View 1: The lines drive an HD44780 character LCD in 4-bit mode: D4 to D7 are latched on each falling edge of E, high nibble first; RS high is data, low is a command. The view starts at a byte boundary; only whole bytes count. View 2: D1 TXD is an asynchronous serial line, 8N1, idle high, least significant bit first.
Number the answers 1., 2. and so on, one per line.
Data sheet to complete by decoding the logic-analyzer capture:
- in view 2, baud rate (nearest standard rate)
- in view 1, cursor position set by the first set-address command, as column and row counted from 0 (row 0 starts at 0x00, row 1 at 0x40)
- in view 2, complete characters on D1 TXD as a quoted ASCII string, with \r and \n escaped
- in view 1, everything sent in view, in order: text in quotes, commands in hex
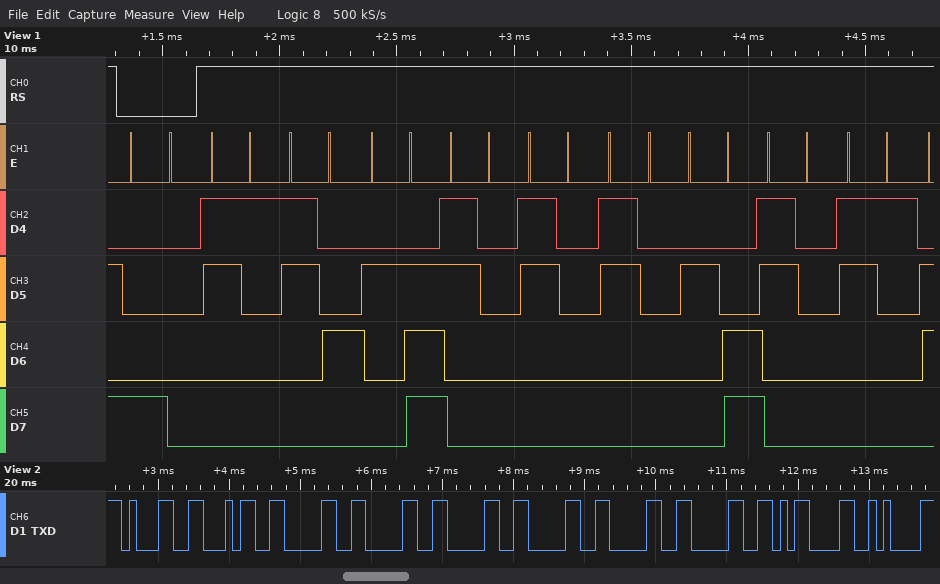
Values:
1. 9600 baud
2. column 0, row 0
3. "14000000\r\n"
4. 0x80 "14.000,01"
